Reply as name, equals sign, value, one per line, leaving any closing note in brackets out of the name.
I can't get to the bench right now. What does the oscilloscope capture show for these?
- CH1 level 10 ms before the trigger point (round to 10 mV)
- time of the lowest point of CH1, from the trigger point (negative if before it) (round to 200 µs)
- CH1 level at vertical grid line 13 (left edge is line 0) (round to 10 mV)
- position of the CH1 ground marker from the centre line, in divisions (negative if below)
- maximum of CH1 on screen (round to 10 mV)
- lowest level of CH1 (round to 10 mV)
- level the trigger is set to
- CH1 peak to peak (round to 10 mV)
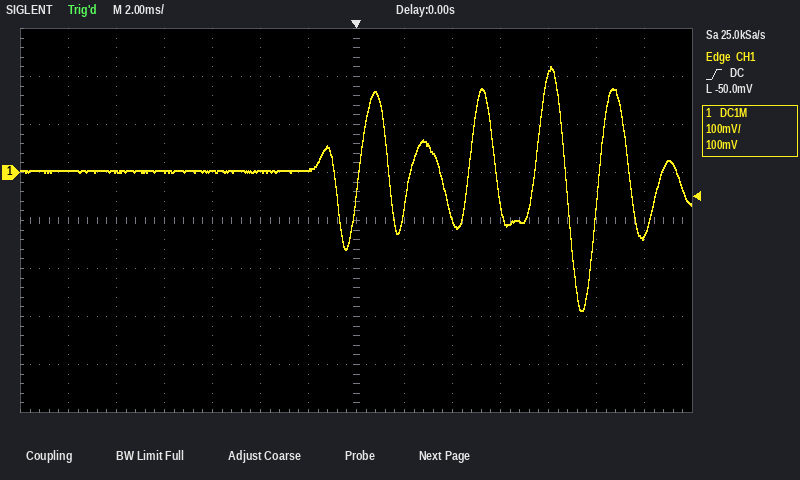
CH1 level 10 ms before the trigger point = 0 mV
time of the lowest point of CH1, from the trigger point (negative if before it) = +9.4 ms
CH1 level at vertical grid line 13 (left edge is line 0) = -130 mV
position of the CH1 ground marker from the centre line, in divisions = +1.0 div
maximum of CH1 on screen = 220 mV
lowest level of CH1 = -290 mV
level the trigger is set to = -50.0 mV
CH1 peak to peak = 510 mV
